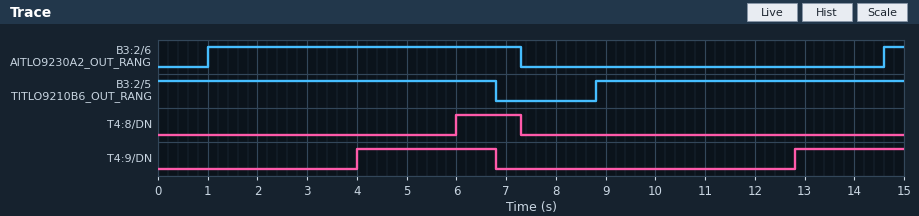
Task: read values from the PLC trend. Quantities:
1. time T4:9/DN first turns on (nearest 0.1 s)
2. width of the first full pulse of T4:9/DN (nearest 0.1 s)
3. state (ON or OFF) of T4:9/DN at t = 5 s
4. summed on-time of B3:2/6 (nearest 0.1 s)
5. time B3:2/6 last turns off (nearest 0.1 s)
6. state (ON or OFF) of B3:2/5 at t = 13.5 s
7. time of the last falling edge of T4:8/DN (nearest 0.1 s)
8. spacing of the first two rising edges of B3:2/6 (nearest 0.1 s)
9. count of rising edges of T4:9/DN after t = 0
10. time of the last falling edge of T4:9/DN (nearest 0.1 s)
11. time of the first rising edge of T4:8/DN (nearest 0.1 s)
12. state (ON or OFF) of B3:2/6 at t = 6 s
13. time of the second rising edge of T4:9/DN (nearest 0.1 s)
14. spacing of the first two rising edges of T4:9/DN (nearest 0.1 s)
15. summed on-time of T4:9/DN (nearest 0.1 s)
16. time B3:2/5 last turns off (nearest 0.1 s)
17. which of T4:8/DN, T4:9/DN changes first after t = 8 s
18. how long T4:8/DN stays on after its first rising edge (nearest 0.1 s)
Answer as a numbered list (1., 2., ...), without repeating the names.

1. 4.0 s
2. 2.8 s
3. ON
4. 6.7 s
5. 7.3 s
6. ON
7. 7.3 s
8. 13.6 s
9. 2
10. 6.8 s
11. 6.0 s
12. ON
13. 12.8 s
14. 8.8 s
15. 5.0 s
16. 6.8 s
17. T4:9/DN
18. 1.3 s
